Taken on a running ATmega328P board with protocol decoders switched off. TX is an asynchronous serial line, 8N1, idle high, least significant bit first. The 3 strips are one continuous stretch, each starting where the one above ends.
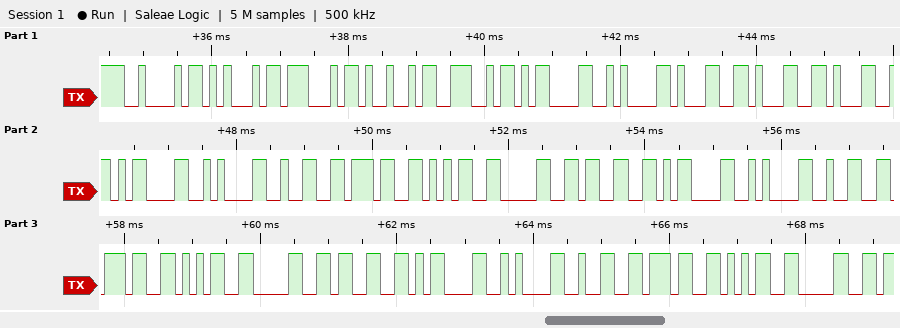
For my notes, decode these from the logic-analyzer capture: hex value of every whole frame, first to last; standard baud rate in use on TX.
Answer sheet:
0x42 0x45 0x47 0x49 0x4E 0x0D 0x0A 0x31 0x31 0x31 0x0D 0x0A 0x32 0x37 0x35 0x30 0x33 0x0D 0x0A 0x32 0x37 0x35 0x30 0x33 0x0D 0x0A 0x32 0x37 0x35 0x30
9600 baud
